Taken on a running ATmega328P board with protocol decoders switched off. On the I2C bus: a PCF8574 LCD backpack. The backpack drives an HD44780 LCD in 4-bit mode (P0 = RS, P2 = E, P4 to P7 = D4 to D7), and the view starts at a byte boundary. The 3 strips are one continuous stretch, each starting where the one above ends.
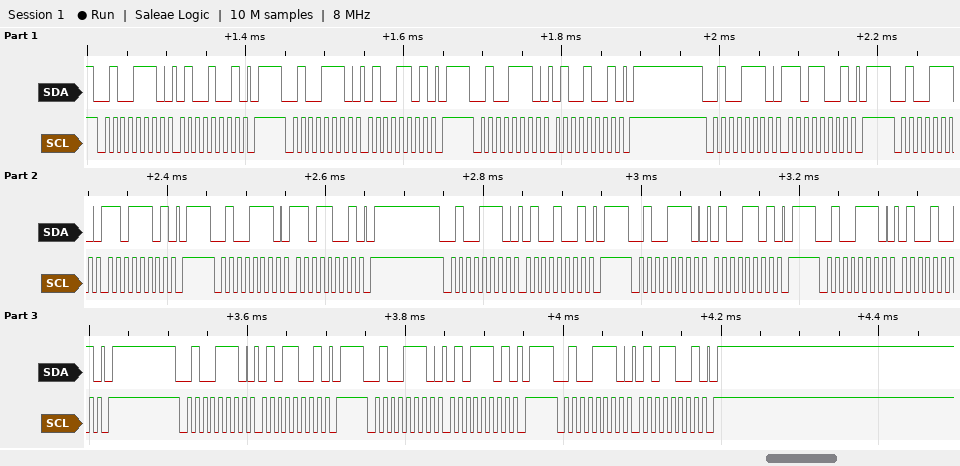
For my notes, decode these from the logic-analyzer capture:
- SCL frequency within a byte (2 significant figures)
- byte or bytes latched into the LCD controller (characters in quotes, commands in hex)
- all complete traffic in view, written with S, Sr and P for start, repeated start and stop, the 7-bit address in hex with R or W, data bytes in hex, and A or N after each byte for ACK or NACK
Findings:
100 kHz
'M' 'E'
S 27W A 49 A P S 27W A 4D A P S 27W A 49 A P S 27W A D9 A P S 27W A DD A P S 27W A D9 A P S 27W A 49 A P S 27W A 4D A P S 27W A 49 A P S 27W A 59 A P S 27W A 5D A P S 27W A 59 A P
